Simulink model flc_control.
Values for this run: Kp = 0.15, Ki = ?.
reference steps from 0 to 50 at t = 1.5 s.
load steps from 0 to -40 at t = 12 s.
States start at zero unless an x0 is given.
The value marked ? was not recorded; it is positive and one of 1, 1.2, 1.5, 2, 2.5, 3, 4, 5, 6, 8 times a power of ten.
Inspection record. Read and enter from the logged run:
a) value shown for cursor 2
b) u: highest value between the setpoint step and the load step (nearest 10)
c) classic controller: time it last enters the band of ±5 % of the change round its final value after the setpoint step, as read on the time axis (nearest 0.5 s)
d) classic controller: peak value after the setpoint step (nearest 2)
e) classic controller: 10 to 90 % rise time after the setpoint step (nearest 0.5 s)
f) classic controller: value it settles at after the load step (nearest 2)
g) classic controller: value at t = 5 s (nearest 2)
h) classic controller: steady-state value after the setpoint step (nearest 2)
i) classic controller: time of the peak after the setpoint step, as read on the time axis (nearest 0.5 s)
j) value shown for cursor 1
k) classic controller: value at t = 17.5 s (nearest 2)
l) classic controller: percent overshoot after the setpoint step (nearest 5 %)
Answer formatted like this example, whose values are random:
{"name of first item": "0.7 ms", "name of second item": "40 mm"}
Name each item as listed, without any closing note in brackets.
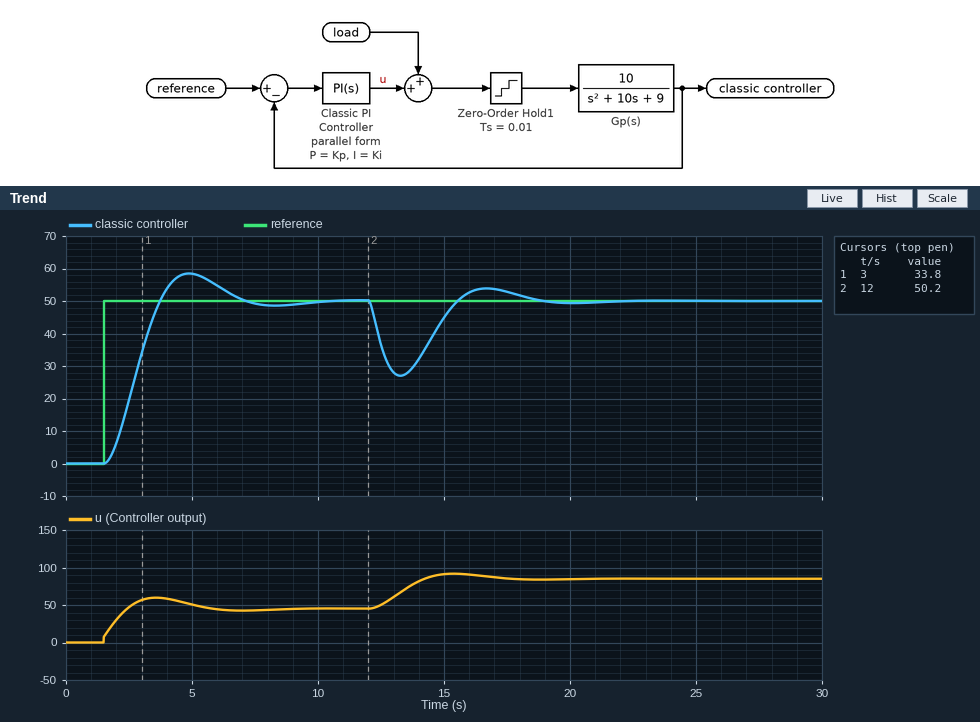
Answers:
{"value shown for cursor 2": "50.2", "u: highest value between the setpoint step and the load step": "60", "classic controller: time it last enters the band of ±5 % of the change round its final value after the setpoint step, as read on the time axis": "6.5 s", "classic controller: peak value after the setpoint step": "58", "classic controller: 10 to 90 % rise time after the setpoint step": "1.5 s", "classic controller: value it settles at after the load step": "50", "classic controller: value at t = 5 s": "58", "classic controller: steady-state value after the setpoint step": "50", "classic controller: time of the peak after the setpoint step, as read on the time axis": "5.0 s", "value shown for cursor 1": "33.8", "classic controller: value at t = 17.5 s": "52", "classic controller: percent overshoot after the setpoint step": "15 %"}
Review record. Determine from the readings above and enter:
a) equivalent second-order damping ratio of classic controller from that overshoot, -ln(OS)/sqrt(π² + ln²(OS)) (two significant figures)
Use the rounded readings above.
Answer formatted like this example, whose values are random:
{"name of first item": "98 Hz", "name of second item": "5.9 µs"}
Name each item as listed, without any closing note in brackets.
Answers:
{"equivalent second-order damping ratio of classic controller from that overshoot, -ln(OS)/sqrt(π² + ln²(OS))": "0.52"}
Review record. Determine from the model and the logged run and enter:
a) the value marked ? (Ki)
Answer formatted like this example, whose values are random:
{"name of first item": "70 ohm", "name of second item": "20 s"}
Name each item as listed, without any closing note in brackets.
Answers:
{"the value marked ?": "1"}
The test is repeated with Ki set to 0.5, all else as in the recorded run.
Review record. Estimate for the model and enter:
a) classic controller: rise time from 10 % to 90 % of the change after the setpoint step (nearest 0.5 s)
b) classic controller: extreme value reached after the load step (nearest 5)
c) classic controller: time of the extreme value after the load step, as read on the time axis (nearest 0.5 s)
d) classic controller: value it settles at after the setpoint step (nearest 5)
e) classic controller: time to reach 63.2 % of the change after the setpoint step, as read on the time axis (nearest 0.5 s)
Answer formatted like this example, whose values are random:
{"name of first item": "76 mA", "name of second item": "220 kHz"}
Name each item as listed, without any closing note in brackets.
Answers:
{"classic controller: rise time from 10 % to 90 % of the change after the setpoint step": "3.0 s", "classic controller: extreme value reached after the load step": "25", "classic controller: time of the extreme value after the load step, as read on the time axis": "13.5 s", "classic controller: value it settles at after the setpoint step": "50", "classic controller: time to reach 63.2 % of the change after the setpoint step, as read on the time axis": "3.5 s"}
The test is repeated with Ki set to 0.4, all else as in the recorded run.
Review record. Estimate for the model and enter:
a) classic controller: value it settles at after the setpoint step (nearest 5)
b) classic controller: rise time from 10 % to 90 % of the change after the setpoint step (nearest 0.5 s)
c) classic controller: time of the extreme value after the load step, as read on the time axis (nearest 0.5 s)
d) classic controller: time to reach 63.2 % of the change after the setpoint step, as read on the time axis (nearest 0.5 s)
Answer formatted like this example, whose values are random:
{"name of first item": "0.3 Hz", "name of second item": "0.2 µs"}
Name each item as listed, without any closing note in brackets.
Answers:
{"classic controller: value it settles at after the setpoint step": "50", "classic controller: rise time from 10 % to 90 % of the change after the setpoint step": "4.0 s", "classic controller: time of the extreme value after the load step, as read on the time axis": "13.5 s", "classic controller: time to reach 63.2 % of the change after the setpoint step, as read on the time axis": "4.0 s"}
